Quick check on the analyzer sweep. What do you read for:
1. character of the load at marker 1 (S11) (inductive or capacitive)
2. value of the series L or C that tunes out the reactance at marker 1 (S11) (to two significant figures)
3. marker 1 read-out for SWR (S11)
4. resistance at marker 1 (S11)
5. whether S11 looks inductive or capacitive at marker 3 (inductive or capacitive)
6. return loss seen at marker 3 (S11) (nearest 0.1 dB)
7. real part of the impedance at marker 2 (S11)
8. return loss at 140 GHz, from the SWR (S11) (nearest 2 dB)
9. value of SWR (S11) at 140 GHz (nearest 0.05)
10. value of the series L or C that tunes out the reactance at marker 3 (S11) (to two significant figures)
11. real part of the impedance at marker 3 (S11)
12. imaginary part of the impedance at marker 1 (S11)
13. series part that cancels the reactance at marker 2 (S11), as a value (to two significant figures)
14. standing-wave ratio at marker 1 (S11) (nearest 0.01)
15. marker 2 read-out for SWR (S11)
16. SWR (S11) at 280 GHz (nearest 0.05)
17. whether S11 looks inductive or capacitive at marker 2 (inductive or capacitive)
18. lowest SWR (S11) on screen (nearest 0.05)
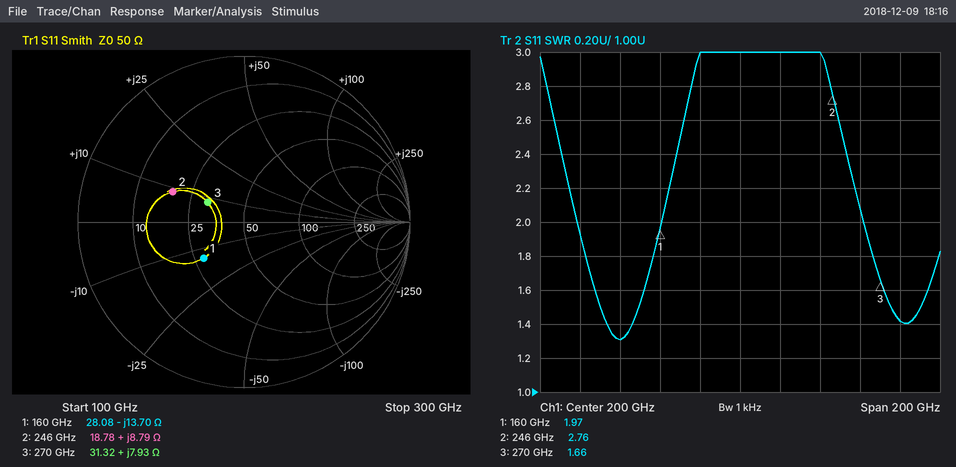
capacitive
14 pH
1.97
28.08 Ω
inductive
12.1 dB
18.78 Ω
18 dB
1.30
74 fF
31.32 Ω
-13.70 Ω
74 fF
1.97
2.76
1.40
inductive
1.30
